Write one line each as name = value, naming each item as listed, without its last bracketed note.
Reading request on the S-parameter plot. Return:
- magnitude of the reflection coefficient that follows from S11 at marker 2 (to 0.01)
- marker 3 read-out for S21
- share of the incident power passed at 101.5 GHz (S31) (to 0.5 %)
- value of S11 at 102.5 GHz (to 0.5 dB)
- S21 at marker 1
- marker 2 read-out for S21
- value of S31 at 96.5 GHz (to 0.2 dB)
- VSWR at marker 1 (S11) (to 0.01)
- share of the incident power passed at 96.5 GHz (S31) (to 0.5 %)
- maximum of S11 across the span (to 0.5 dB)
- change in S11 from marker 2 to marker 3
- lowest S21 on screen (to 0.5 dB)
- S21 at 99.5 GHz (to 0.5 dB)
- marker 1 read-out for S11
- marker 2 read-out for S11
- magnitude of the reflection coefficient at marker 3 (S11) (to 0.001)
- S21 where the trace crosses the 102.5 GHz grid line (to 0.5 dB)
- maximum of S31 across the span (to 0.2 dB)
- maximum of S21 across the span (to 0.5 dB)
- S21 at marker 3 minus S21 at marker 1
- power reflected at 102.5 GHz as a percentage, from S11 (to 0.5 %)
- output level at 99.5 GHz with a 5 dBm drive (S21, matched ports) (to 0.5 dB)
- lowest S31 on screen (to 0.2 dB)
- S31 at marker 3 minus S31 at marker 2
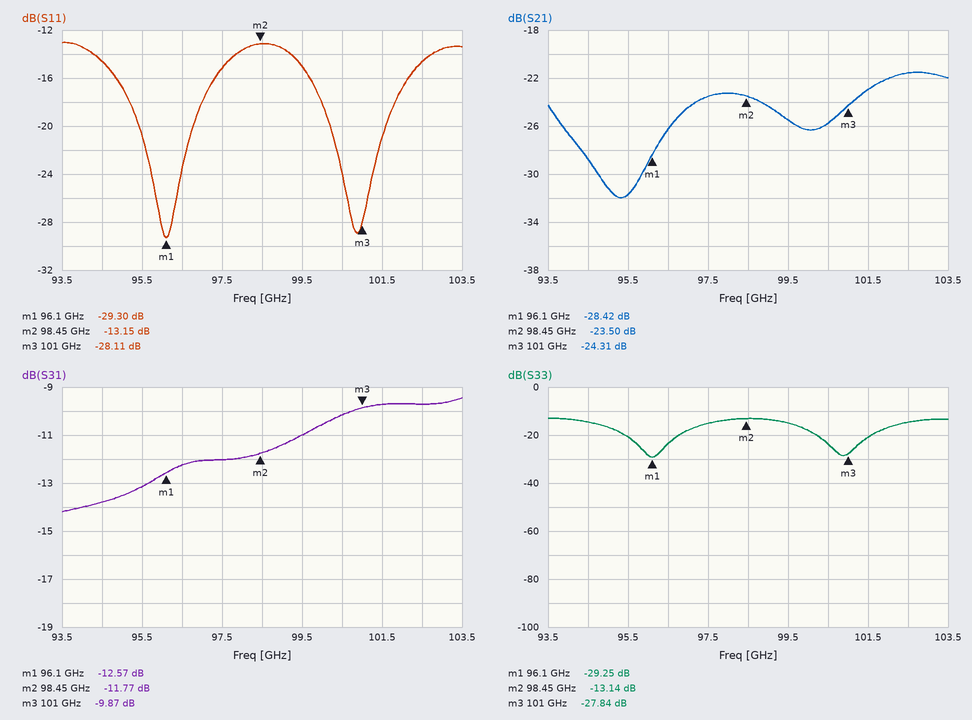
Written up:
magnitude of the reflection coefficient that follows from S11 at marker 2 = 0.22
marker 3 read-out for S21 = -24.31 dB
share of the incident power passed at 101.5 GHz (S31) = 10.5 %
value of S11 at 102.5 GHz = -14.5 dB
S21 at marker 1 = -28.42 dB
marker 2 read-out for S21 = -23.50 dB
value of S31 at 96.5 GHz = -12.2 dB
VSWR at marker 1 (S11) = 1.07
share of the incident power passed at 96.5 GHz (S31) = 6.0 %
maximum of S11 across the span = -13.0 dB
change in S11 from marker 2 to marker 3 = -14.96 dB
lowest S21 on screen = -32.0 dB
S21 at 99.5 GHz = -25.5 dB
marker 1 read-out for S11 = -29.30 dB
marker 2 read-out for S11 = -13.15 dB
magnitude of the reflection coefficient at marker 3 (S11) = 0.039
S21 where the trace crosses the 102.5 GHz grid line = -21.5 dB
maximum of S31 across the span = -9.4 dB
maximum of S21 across the span = -21.5 dB
S21 at marker 3 minus S21 at marker 1 = 4.11 dB
power reflected at 102.5 GHz as a percentage, from S11 = 3.5 %
output level at 99.5 GHz with a 5 dBm drive (S21, matched ports) = -20.5 dBm
lowest S31 on screen = -14.2 dB
S31 at marker 3 minus S31 at marker 2 = 1.90 dB
